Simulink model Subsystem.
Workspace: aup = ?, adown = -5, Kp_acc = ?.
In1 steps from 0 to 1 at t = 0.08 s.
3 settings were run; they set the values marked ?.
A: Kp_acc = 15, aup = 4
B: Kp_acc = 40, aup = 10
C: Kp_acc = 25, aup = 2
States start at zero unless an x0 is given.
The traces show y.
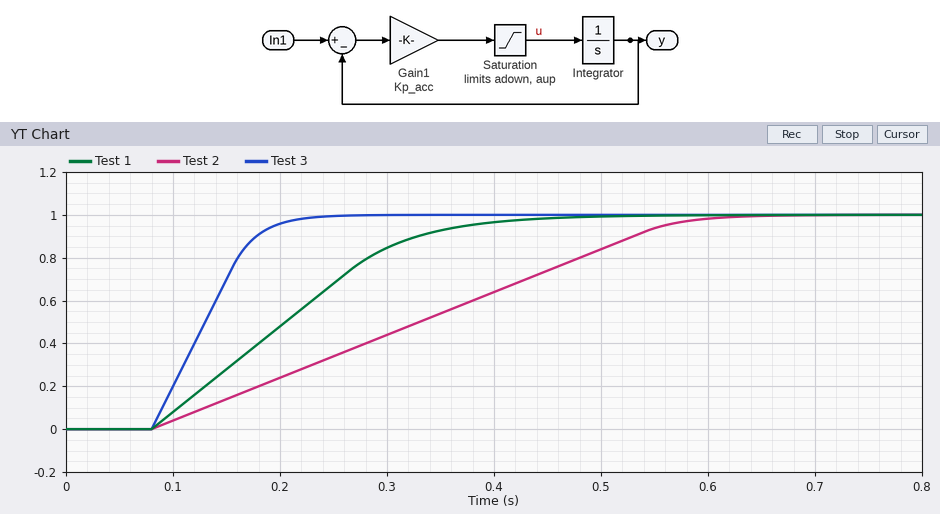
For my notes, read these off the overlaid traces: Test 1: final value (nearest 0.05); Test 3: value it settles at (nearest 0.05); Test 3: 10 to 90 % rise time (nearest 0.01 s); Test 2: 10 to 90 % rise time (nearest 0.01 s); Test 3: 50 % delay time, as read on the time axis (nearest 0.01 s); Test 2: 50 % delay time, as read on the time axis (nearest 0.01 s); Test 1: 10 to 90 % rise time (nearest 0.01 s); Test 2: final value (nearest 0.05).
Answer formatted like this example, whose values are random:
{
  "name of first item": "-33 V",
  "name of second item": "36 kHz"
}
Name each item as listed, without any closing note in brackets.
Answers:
{
  "Test 1: final value": "1.00",
  "Test 3: value it settles at": "1.00",
  "Test 3: 10 to 90 % rise time": "0.09 s",
  "Test 2: 10 to 90 % rise time": "0.40 s",
  "Test 3: 50 % delay time, as read on the time axis": "0.13 s",
  "Test 2: 50 % delay time, as read on the time axis": "0.33 s",
  "Test 1: 10 to 90 % rise time": "0.22 s",
  "Test 2: final value": "1.00"
}
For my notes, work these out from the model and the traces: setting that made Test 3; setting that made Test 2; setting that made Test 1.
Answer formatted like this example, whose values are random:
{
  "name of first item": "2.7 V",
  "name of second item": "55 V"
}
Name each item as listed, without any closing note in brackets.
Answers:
{
  "setting that made Test 3": "B",
  "setting that made Test 2": "C",
  "setting that made Test 1": "A"
}
